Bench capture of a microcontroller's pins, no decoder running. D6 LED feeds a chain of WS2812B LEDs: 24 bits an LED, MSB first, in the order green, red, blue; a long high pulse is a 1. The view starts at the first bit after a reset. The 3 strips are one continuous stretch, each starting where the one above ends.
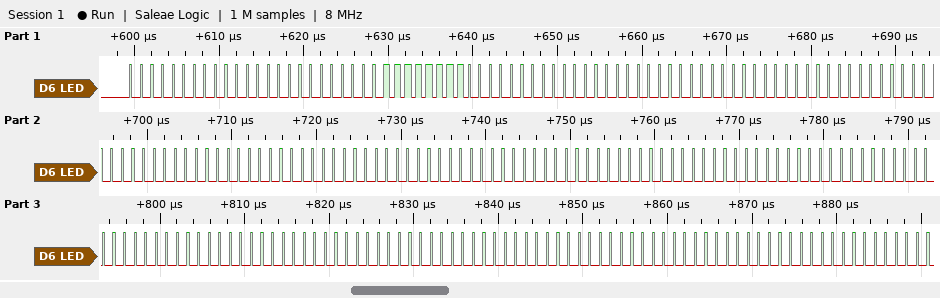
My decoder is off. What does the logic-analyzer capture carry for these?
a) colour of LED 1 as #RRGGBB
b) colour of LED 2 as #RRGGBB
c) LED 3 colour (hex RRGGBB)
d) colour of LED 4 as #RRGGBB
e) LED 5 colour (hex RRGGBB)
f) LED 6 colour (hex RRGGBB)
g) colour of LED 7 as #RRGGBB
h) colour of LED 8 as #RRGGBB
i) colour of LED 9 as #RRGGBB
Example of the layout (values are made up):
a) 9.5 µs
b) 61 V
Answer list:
a) #000000
b) #00FF00
c) #000000
d) #000000
e) #000000
f) #000000
g) #000000
h) #000000
i) #000000
